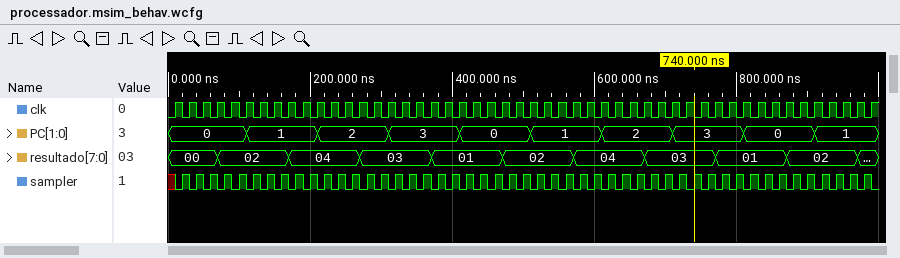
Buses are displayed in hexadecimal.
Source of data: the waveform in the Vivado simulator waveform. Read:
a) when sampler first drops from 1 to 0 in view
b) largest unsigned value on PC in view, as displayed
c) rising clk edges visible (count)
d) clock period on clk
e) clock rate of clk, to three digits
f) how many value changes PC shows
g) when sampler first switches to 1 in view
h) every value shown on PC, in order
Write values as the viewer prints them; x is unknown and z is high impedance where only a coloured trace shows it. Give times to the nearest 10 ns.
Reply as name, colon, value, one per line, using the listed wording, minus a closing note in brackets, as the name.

when sampler first drops from 1 to 0 in view: 30 ns
largest unsigned value on PC in view, as displayed: 3
rising clk edges visible: 50
clock period on clk: 20 ns
clock rate of clk, to three digits: 50.0 MHz
how many value changes PC shows: 9
when sampler first switches to 1 in view: 20 ns
every value shown on PC, in order: 0, 1, 2, 3, 0, 1, 2, 3, 0, 1
